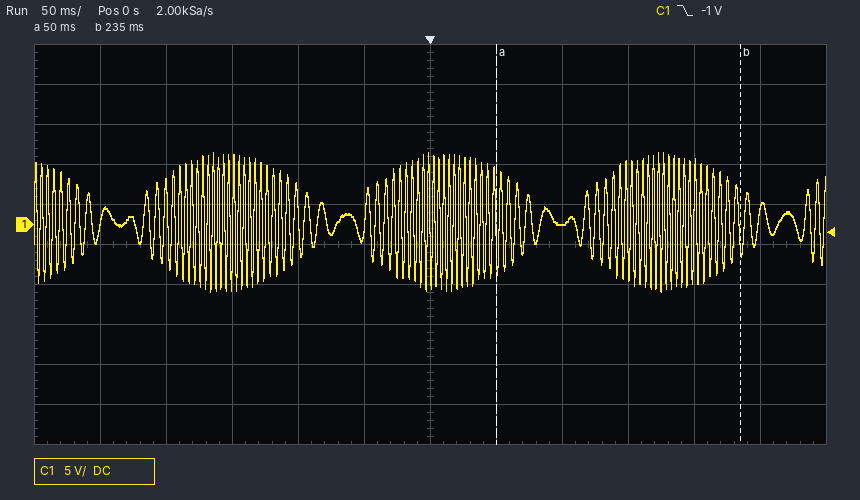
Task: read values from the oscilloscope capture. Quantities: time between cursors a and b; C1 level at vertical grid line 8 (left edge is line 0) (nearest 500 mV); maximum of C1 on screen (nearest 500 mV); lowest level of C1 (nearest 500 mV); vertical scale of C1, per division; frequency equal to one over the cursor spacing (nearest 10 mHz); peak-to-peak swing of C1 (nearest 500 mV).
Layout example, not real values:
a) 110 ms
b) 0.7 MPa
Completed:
a) 185 ms
b) 0.0 V
c) 9.0 V
d) -8.5 V
e) 5 V
f) 5.41 Hz
g) 17.5 V
